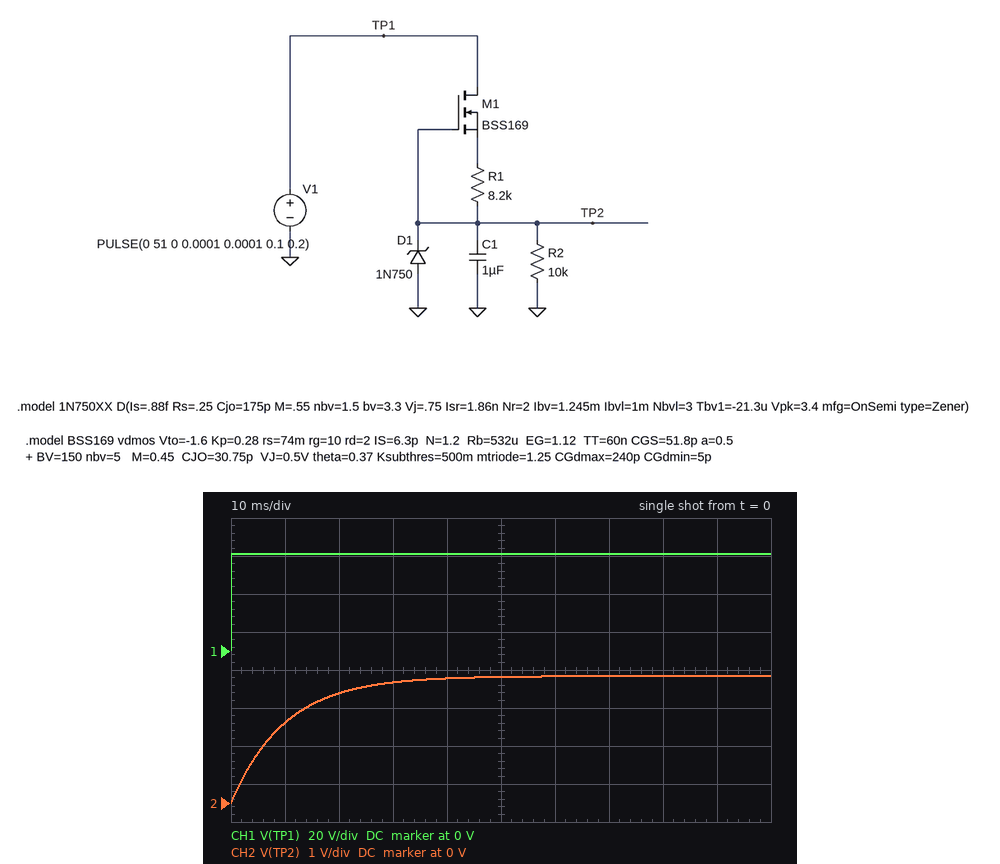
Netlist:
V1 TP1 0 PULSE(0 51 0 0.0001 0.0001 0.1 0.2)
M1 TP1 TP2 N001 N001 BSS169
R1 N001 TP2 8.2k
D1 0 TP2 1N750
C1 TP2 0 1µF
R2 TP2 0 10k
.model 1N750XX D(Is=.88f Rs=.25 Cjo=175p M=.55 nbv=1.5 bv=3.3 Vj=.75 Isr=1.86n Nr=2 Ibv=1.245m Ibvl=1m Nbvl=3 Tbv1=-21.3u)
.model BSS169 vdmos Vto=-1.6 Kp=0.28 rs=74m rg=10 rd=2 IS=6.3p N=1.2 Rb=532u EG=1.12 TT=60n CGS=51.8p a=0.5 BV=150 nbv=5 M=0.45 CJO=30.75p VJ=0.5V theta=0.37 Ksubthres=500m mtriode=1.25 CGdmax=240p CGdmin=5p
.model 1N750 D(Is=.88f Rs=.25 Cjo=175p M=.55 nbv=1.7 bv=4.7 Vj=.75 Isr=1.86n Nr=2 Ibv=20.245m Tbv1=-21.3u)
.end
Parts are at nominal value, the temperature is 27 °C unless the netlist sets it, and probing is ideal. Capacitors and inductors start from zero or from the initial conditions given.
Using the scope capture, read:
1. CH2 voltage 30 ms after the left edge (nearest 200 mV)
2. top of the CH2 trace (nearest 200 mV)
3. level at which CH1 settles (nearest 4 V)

3.2 V
3.4 V
52 V
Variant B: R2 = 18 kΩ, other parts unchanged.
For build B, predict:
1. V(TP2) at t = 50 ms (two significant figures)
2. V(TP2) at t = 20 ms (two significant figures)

4.5 V
4.0 V
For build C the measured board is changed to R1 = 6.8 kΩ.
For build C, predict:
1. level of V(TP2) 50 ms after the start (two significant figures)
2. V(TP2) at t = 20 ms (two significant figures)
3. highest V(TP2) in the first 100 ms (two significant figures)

3.9 V
3.4 V
4.0 V
